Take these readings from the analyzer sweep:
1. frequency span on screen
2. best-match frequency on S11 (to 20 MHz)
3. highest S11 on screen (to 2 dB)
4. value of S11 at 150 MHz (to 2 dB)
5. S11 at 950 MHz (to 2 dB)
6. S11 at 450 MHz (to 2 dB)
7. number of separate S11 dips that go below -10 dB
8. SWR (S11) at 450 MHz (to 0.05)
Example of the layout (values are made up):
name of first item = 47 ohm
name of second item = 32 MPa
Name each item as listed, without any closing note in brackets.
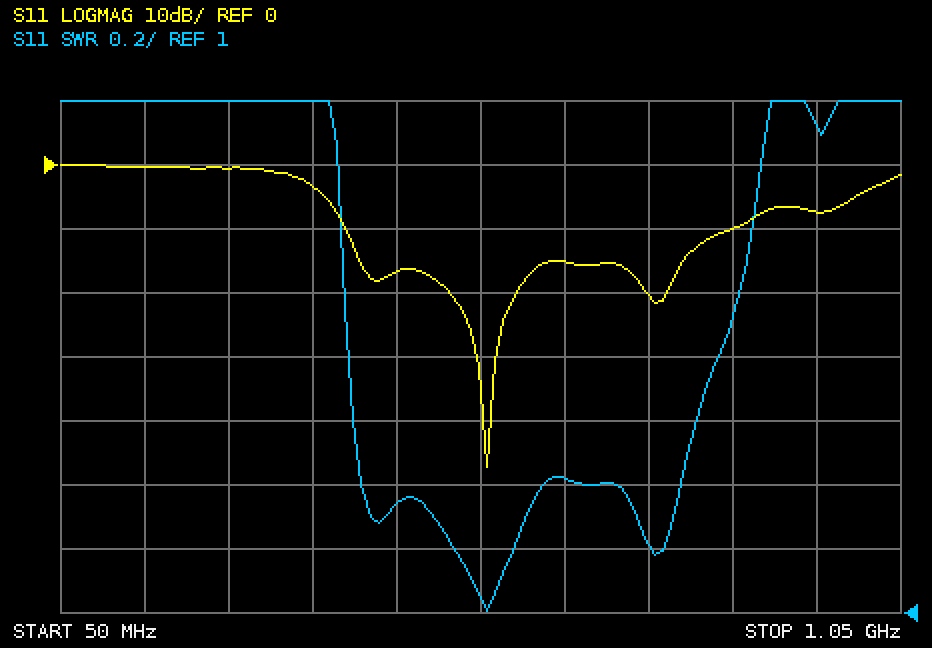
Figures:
frequency span on screen = 1 GHz
best-match frequency on S11 = 560 MHz
highest S11 on screen = 0 dB
value of S11 at 150 MHz = 0 dB
S11 at 950 MHz = -8 dB
S11 at 450 MHz = -16 dB
number of separate S11 dips that go below -10 dB = 2
SWR (S11) at 450 MHz = 1.35
